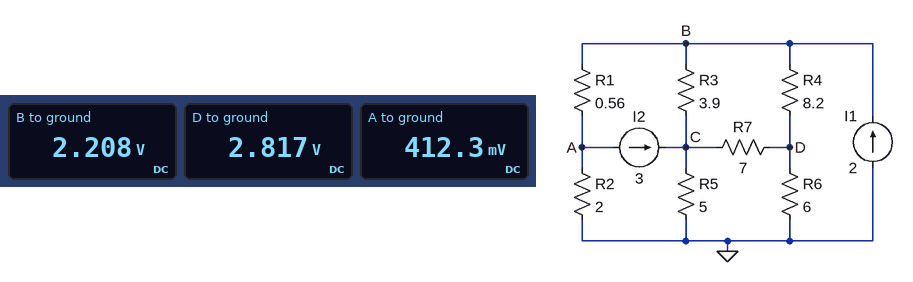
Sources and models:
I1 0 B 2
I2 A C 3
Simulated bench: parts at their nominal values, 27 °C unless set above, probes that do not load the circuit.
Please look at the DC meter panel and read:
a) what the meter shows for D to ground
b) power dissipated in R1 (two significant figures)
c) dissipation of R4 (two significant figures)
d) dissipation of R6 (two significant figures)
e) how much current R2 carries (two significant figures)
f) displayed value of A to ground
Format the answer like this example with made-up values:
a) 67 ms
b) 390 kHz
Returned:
a) 2.817 V
b) 5.8 W
c) 45 mW
d) 1.3 W
e) 210 mA
f) 412.3 mV
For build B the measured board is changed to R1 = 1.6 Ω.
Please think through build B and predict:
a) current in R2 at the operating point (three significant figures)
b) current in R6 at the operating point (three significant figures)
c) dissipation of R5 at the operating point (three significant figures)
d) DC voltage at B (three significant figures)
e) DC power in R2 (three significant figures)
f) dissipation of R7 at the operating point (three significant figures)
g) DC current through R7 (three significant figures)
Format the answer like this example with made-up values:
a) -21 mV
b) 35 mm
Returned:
a) 163 mA
b) 623 mA
c) 11.9 W
d) 4.21 V
e) 53.3 mW
f) 2.24 W
g) 566 mA
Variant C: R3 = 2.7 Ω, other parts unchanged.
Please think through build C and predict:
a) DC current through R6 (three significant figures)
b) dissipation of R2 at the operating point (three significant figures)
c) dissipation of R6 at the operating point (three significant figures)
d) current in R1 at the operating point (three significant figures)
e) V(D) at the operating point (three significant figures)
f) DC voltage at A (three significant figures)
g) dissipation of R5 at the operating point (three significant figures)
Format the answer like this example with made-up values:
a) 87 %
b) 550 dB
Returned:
a) 454 mA
b) 221 mW
c) 1.24 W
d) 3.33 A
e) 2.72 V
f) 665 mV
g) 7.36 W
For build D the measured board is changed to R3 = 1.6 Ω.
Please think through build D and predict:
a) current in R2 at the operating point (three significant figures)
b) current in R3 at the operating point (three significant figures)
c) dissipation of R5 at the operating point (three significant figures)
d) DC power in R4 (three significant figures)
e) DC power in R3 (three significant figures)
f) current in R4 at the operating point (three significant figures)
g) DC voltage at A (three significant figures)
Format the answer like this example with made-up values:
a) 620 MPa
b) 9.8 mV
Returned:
a) 489 mA
b) 1.53 A
c) 5.79 W
d) 12.7 mW
e) 3.74 W
f) 39.4 mA
g) 979 mV
